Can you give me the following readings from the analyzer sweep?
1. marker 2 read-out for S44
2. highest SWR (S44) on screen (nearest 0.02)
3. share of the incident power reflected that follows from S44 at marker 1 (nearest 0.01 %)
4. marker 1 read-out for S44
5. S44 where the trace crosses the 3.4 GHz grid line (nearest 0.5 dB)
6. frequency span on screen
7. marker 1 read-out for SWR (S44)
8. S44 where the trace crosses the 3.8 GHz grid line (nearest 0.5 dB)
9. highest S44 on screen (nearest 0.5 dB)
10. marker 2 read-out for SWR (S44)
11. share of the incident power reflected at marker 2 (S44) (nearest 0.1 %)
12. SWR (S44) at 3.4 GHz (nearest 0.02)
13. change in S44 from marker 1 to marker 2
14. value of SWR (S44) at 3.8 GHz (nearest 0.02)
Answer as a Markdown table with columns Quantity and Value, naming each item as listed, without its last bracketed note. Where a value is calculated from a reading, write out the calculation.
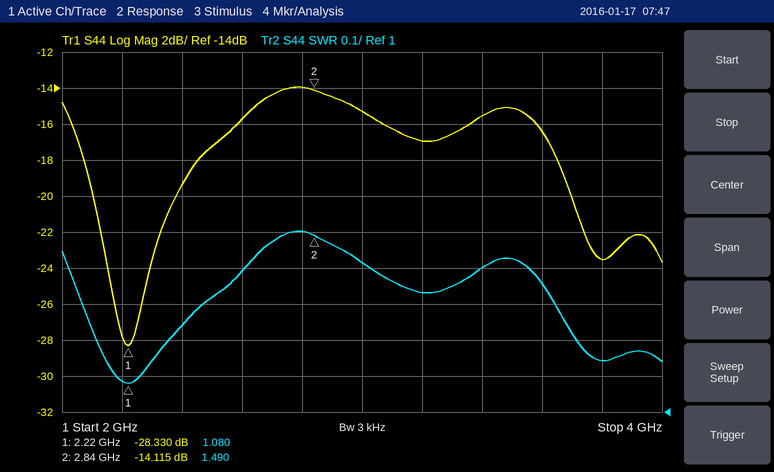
| Quantity | Value |
|---|---|
| marker 2 read-out for S44 | -14.115 dB |
| highest SWR (S44) on screen | 1.50 |
| share of the incident power reflected that follows from S44 at marker 1 | 10^(-28.33/10) ≈ 0.15 % |
| marker 1 read-out for S44 | -28.330 dB |
| S44 where the trace crosses the 3.4 GHz grid line | -15.5 dB |
| frequency span on screen | 2 GHz |
| marker 1 read-out for SWR | 1.080 |
| S44 where the trace crosses the 3.8 GHz grid line | -23.5 dB |
| highest S44 on screen | -14.0 dB |
| marker 2 read-out for SWR | 1.490 |
| share of the incident power reflected at marker 2 (S44) | 10^(-14.115/10) ≈ 3.9 % |
| SWR (S44) at 3.4 GHz | 1.40 |
| change in S44 from marker 1 to marker 2 | -14.115 − (-28.33) = 14.215 dB |
| value of SWR (S44) at 3.8 GHz | 1.14 |
